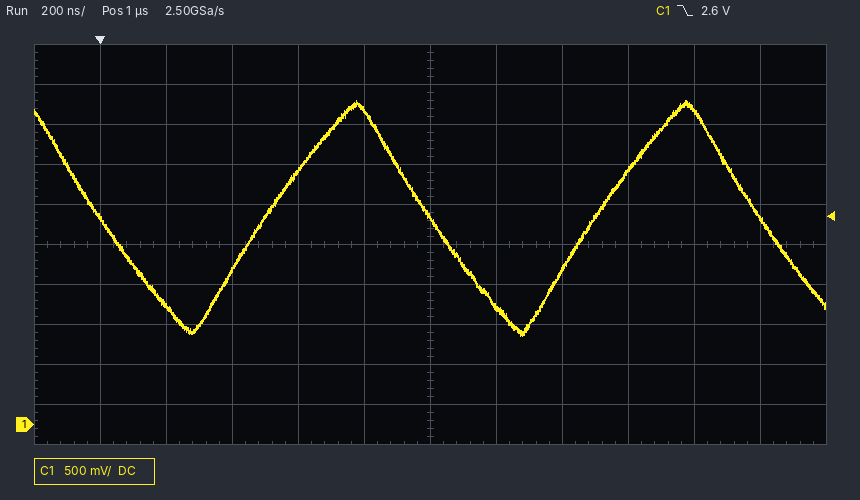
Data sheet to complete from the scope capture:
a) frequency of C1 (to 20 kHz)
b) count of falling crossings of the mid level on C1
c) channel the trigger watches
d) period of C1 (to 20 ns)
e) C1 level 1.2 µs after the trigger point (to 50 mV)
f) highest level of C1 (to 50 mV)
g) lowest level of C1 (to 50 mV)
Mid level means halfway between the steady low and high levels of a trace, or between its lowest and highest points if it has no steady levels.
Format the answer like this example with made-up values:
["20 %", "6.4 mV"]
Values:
["1.00 MHz", "3", "C1", "1.00 µs", "1.45 V", "4.05 V", "1.10 V"]
